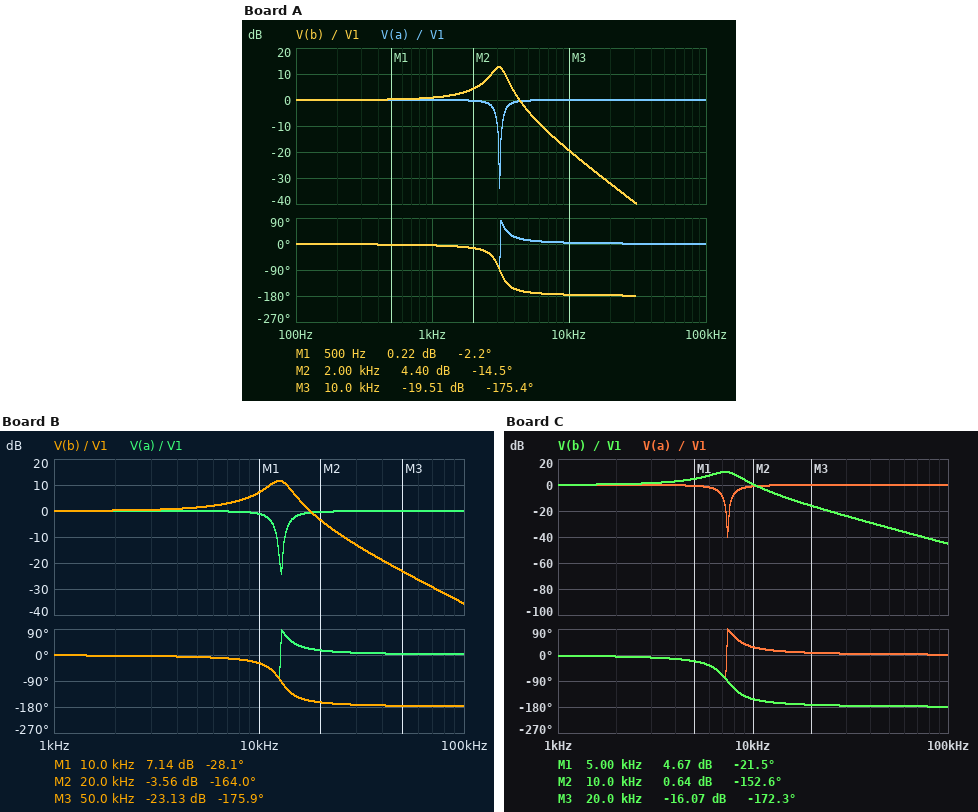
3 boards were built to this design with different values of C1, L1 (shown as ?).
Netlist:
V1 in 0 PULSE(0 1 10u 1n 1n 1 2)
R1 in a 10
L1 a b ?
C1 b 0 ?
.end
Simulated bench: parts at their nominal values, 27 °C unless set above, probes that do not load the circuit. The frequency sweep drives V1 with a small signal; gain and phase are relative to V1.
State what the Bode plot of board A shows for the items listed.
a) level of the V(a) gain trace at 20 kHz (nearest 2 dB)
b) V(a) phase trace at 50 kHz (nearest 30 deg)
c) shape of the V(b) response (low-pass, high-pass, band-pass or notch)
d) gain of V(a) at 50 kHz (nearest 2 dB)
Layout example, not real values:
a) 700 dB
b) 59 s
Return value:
a) 0 dB
b) 0 deg
c) low-pass
d) 0 dB
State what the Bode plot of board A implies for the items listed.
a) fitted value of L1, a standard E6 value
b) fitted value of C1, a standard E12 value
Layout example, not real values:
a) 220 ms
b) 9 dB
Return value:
a) 2.2 mH
b) 1.2 µF
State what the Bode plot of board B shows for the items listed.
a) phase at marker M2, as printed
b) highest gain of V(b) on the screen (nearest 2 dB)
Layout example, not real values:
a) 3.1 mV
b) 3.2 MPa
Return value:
a) -164.0 deg
b) 12 dB
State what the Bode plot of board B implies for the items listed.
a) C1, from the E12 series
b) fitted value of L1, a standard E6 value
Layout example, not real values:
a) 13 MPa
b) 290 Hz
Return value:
a) 330 nF
b) 470 µH
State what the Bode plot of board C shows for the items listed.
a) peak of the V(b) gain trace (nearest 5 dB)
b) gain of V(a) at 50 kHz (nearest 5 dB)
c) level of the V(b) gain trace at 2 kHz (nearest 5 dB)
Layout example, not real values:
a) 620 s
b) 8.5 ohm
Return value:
a) 10 dB
b) 0 dB
c) 0 dB
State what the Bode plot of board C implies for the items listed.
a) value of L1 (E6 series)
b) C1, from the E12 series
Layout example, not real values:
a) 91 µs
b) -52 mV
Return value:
a) 680 µH
b) 680 nF
